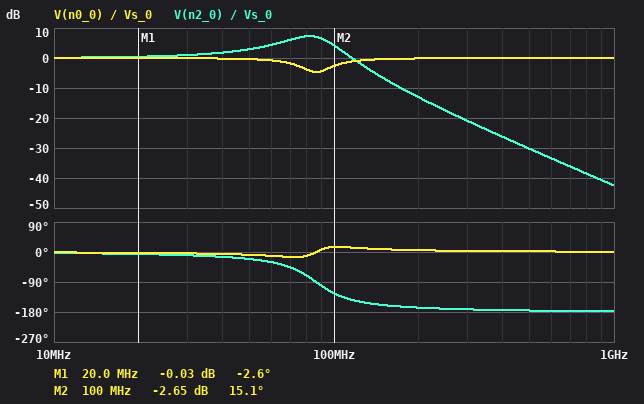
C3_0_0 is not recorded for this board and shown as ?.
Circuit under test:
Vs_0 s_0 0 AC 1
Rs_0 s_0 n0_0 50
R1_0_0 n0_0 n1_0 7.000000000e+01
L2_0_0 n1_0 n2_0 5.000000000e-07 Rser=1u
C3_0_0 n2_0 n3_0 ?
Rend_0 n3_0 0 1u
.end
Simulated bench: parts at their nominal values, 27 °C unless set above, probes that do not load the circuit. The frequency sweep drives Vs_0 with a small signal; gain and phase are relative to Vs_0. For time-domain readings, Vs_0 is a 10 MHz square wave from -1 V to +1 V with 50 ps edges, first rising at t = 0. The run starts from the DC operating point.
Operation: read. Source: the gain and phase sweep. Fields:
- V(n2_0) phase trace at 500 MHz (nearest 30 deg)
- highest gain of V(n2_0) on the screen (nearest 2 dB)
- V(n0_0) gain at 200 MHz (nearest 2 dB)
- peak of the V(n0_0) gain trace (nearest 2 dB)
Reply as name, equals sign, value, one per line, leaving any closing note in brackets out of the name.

V(n2_0) phase trace at 500 MHz = -180 deg
highest gain of V(n2_0) on the screen = 8 dB
V(n0_0) gain at 200 MHz = 0 dB
peak of the V(n0_0) gain trace = 0 dB
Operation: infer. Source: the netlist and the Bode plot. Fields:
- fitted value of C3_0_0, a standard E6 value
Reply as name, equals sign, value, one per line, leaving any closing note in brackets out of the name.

fitted value of C3_0_0, a standard E6 value = 6.8 pF
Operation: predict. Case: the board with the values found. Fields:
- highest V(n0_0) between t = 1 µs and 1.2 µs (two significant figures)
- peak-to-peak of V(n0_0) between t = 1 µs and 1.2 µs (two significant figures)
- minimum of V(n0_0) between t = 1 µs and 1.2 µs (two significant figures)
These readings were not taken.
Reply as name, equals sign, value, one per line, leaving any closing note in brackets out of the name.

highest V(n0_0) between t = 1 µs and 1.2 µs = 1.1 V
peak-to-peak of V(n0_0) between t = 1 µs and 1.2 µs = 2.3 V
minimum of V(n0_0) between t = 1 µs and 1.2 µs = -1.1 V
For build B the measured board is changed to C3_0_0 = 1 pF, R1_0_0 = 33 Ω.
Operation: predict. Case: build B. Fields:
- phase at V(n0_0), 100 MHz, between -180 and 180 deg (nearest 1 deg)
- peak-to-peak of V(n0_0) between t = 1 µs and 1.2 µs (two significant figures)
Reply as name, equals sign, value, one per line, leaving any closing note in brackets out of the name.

phase at V(n0_0), 100 MHz, between -180 and 180 deg = -2 deg
peak-to-peak of V(n0_0) between t = 1 µs and 1.2 µs = 2.2 V
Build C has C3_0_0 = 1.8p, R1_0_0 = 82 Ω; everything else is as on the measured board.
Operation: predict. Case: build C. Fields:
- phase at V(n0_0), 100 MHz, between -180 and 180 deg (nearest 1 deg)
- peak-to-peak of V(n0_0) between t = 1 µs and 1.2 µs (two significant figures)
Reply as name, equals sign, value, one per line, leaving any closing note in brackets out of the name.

phase at V(n0_0), 100 MHz, between -180 and 180 deg = -5 deg
peak-to-peak of V(n0_0) between t = 1 µs and 1.2 µs = 2.2 V
